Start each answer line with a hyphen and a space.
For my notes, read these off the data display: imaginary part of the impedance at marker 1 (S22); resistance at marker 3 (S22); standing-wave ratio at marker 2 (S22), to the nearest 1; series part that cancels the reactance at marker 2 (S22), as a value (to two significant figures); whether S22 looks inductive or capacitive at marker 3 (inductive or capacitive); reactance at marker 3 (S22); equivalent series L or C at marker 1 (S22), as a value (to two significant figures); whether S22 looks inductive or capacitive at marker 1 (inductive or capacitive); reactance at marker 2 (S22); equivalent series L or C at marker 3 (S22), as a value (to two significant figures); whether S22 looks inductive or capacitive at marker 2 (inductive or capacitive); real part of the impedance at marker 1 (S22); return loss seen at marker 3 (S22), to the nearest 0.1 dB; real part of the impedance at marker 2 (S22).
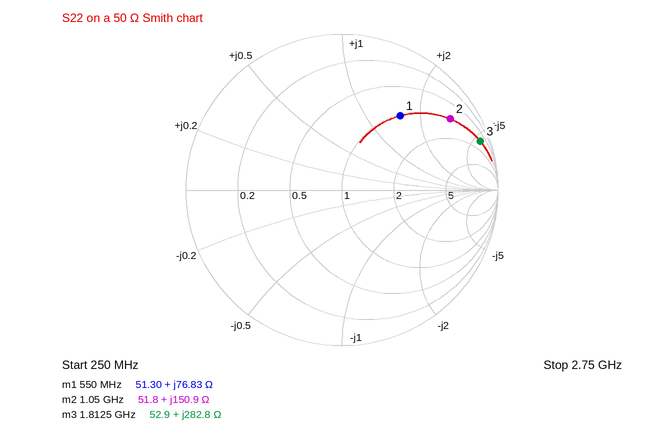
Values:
- +76.83 Ω
- 52.9 Ω
- 11
- 1.0 pF
- inductive
- +282.8 Ω
- 22 nH
- inductive
- +150.9 Ω
- 25 nH
- inductive
- 51.30 Ω
- 0.5 dB
- 51.8 Ω
